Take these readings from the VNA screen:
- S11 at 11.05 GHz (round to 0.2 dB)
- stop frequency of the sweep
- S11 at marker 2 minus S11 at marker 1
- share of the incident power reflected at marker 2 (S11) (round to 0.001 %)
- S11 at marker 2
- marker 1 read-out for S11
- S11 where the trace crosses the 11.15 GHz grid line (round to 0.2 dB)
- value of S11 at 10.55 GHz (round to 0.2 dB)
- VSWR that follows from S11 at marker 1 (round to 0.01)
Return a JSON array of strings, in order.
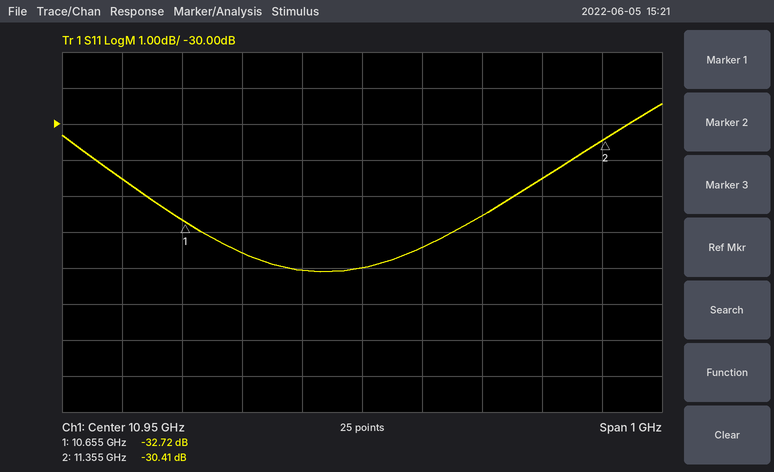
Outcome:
["-33.4 dB", "11.45 GHz", "2.31 dB", "0.091 %", "-30.41 dB", "-32.72 dB", "-32.6 dB", "-31.6 dB", "1.05"]
